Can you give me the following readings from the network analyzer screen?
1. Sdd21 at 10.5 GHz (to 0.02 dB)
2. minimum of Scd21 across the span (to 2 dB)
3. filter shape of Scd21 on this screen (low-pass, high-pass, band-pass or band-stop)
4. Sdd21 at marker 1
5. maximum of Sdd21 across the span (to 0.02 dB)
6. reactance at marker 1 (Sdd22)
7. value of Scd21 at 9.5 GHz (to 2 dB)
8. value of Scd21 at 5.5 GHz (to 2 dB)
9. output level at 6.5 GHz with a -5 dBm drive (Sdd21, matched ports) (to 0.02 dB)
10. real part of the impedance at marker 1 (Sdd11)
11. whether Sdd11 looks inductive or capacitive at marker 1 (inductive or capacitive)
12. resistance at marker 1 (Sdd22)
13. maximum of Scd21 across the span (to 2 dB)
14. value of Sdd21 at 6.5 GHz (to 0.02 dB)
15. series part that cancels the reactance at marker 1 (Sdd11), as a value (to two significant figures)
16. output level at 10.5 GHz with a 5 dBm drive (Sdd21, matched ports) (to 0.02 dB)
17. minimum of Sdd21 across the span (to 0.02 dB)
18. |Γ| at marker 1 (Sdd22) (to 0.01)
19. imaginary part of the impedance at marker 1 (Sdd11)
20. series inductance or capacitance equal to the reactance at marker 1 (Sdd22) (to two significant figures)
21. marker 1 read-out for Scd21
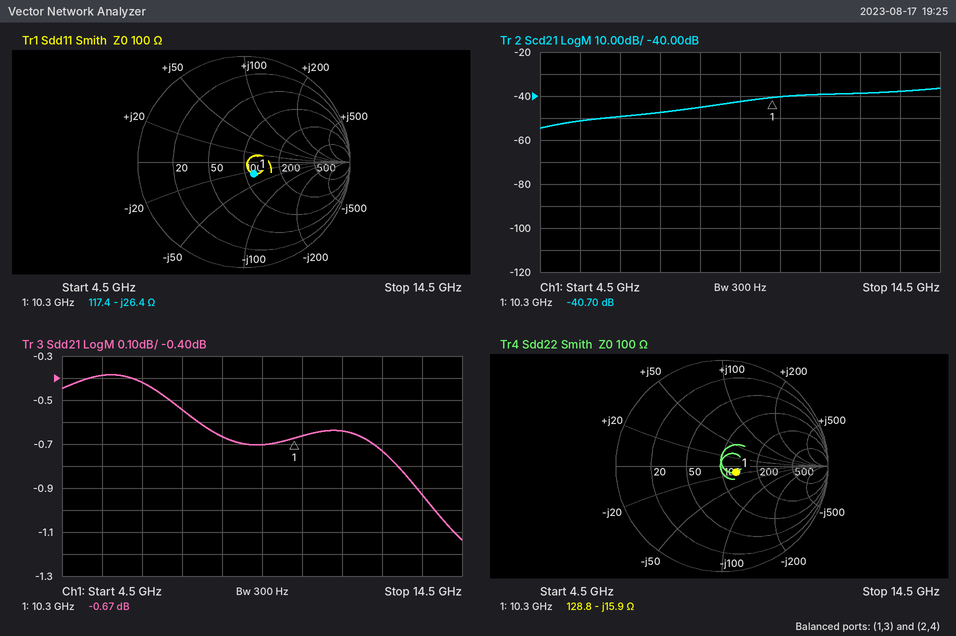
-0.66 dB
-54 dB
high-pass
-0.67 dB
-0.38 dB
-15.9 Ω
-42 dB
-52 dB
-5.42 dBm
117.4 Ω
capacitive
128.8 Ω
-36 dB
-0.42 dB
410 pH
4.34 dBm
-1.14 dB
0.14
-26.4 Ω
970 fF
-40.70 dB
